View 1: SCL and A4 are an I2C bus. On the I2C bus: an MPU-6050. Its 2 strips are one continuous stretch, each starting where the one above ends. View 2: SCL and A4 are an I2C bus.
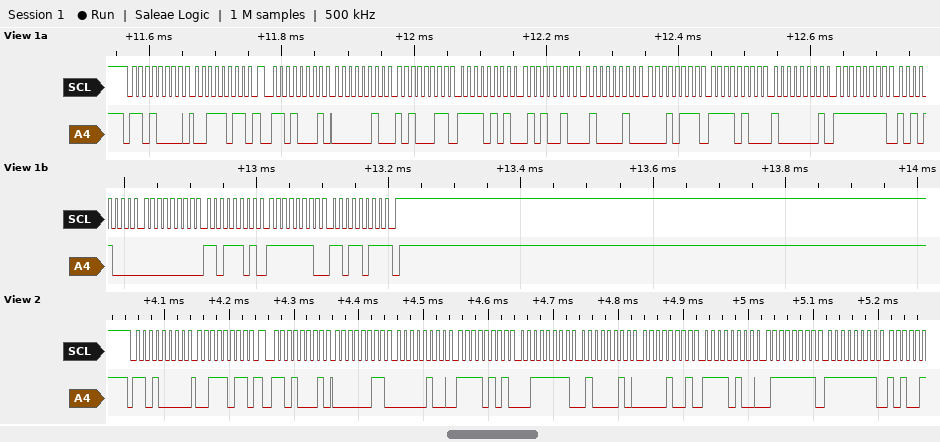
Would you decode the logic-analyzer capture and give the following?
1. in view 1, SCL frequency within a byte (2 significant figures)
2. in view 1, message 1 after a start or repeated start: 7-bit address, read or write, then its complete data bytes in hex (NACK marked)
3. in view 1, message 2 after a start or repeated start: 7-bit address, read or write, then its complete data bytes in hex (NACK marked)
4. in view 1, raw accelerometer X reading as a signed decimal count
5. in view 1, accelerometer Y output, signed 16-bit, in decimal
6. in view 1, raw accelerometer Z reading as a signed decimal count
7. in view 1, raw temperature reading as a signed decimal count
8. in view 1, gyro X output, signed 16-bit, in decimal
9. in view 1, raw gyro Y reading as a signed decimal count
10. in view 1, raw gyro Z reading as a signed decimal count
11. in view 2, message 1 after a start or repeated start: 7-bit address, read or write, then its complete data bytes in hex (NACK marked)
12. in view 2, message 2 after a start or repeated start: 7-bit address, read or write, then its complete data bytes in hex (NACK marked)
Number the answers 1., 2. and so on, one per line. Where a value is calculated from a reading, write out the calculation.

1. 100 kHz
2. 0x68 write: 3B
3. 0x68 read: 02 A3 F5 52 42 17 F4 81 FF A8 00 DD FE DB NACK
4. 0x02A3 = 675
5. 0xF552 = -2734
6. 0x4217 = 16919
7. 0xF481 = -2943
8. 0xFFA8 = -88
9. 0x00DD = 221
10. 0xFEDB = -293
11. 0x68 write: 3B
12. 0x68 read: 03 04 F5 3F 42 09 F4 7F FF
